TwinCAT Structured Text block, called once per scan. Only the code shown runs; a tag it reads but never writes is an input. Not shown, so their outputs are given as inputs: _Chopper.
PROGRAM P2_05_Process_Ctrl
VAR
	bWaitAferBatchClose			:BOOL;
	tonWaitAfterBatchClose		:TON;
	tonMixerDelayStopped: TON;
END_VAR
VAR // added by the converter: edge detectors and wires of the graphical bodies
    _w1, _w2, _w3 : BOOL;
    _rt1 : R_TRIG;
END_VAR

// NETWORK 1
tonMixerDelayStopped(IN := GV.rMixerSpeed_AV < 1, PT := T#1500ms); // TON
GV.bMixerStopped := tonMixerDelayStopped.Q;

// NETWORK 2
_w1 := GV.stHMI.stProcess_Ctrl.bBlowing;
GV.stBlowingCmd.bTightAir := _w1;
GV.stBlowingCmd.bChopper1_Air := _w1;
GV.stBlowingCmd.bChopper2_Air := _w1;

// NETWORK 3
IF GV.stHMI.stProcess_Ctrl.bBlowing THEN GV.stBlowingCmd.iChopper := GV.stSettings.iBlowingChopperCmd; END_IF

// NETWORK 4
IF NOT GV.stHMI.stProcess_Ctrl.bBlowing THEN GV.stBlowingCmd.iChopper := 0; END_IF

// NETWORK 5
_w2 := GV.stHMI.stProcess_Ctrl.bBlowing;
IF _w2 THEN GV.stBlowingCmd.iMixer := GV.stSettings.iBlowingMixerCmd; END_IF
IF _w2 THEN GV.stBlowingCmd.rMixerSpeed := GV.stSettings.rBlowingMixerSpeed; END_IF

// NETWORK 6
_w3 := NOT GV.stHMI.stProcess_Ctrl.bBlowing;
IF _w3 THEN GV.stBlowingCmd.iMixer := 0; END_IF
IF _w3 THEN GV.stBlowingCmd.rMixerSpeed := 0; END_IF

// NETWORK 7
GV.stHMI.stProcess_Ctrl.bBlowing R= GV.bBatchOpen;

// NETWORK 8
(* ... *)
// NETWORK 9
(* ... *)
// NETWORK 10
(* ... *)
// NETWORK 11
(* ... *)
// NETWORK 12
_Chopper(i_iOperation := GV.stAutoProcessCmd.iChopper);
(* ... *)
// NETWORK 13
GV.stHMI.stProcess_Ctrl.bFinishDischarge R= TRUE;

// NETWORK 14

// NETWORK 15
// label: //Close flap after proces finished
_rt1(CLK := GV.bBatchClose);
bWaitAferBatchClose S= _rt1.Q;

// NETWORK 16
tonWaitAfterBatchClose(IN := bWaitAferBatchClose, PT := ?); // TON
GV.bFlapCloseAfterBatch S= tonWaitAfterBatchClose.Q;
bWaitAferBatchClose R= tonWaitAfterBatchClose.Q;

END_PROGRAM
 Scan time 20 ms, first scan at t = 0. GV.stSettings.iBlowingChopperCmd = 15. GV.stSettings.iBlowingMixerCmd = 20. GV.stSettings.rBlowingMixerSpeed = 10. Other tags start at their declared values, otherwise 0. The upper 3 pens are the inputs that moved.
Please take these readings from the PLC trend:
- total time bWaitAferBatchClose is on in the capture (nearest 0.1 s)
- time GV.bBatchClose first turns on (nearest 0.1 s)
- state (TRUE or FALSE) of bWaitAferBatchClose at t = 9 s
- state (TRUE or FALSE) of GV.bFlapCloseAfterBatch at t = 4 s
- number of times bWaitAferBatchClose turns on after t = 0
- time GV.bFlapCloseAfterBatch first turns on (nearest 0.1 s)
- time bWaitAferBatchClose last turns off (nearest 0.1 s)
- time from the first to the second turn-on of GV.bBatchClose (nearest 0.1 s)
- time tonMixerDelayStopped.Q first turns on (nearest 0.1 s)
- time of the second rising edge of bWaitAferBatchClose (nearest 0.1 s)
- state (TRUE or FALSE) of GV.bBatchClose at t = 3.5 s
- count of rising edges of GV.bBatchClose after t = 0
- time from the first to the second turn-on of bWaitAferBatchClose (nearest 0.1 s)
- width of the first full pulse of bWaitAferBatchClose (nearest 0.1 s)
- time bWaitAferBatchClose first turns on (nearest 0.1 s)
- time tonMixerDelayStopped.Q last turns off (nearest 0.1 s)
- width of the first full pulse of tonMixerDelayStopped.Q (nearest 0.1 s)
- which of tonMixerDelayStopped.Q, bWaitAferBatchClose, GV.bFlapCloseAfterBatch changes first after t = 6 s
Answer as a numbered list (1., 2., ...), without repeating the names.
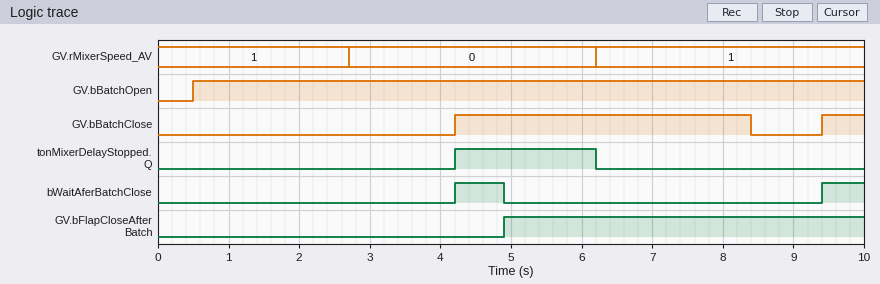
1. 1.3 s
2. 4.2 s
3. FALSE
4. FALSE
5. 2
6. 4.9 s
7. 4.9 s
8. 5.2 s
9. 4.2 s
10. 9.4 s
11. FALSE
12. 2
13. 5.2 s
14. 0.7 s
15. 4.2 s
16. 6.2 s
17. 2.0 s
18. tonMixerDelayStopped.Q
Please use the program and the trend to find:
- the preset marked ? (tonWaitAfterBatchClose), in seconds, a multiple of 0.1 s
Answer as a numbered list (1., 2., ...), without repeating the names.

1. 0.7 s
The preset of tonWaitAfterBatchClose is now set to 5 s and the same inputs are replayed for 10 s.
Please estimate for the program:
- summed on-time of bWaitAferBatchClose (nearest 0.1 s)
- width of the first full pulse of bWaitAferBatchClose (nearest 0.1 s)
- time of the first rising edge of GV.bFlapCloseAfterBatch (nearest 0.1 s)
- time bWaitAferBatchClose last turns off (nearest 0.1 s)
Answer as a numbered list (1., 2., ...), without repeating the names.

1. 5.6 s
2. 5.0 s
3. 9.2 s
4. 9.2 s
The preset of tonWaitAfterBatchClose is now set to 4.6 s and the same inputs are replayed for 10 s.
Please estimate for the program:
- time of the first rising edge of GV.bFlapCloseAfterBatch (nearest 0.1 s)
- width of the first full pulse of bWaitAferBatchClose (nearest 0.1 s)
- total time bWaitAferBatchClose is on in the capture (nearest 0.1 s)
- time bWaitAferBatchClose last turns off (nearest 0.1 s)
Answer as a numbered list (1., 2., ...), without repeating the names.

1. 8.8 s
2. 4.6 s
3. 5.2 s
4. 8.8 s
